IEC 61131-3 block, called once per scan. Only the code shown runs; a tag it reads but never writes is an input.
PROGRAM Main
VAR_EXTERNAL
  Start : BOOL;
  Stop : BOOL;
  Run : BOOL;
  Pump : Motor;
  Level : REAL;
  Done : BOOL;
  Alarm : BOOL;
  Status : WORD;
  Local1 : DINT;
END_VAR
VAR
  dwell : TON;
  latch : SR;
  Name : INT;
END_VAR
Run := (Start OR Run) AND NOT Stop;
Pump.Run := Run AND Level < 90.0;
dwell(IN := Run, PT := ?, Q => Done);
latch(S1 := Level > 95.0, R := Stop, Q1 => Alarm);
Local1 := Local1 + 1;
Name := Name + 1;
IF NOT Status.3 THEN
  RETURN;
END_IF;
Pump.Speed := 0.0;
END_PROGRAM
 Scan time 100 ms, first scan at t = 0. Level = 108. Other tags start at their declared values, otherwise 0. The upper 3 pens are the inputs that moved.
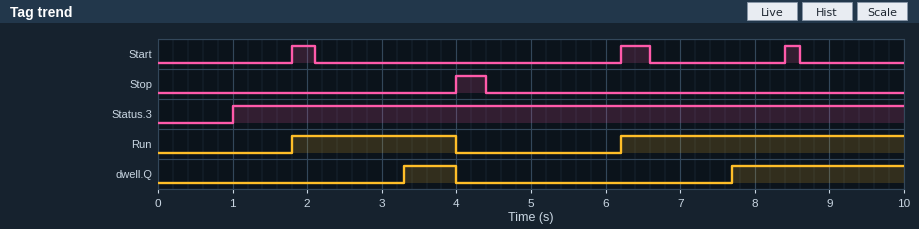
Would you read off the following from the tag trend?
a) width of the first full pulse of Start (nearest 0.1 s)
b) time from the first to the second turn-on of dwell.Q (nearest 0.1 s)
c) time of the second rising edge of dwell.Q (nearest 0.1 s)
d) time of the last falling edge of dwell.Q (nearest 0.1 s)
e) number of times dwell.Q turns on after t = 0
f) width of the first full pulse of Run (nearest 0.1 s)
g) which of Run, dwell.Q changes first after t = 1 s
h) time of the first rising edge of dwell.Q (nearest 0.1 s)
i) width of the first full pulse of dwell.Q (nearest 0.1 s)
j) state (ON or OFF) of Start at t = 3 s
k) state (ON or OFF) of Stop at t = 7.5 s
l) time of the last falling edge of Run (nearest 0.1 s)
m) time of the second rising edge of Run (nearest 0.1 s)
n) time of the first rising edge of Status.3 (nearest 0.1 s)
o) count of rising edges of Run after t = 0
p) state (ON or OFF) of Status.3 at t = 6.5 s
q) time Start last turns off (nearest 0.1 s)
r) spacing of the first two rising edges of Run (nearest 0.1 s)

0.3 s
4.4 s
7.7 s
4.0 s
2
2.2 s
Run
3.3 s
0.7 s
OFF
OFF
4.0 s
6.2 s
1.0 s
2
ON
8.6 s
4.4 s
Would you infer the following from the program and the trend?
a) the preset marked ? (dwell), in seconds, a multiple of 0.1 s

1.5 s
